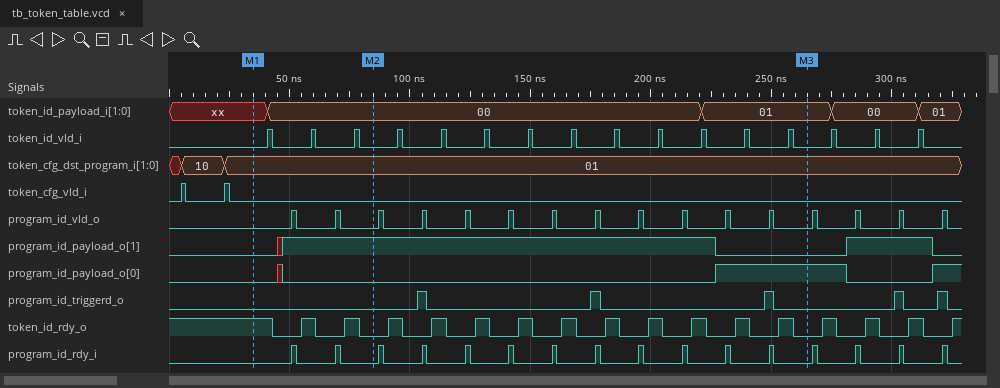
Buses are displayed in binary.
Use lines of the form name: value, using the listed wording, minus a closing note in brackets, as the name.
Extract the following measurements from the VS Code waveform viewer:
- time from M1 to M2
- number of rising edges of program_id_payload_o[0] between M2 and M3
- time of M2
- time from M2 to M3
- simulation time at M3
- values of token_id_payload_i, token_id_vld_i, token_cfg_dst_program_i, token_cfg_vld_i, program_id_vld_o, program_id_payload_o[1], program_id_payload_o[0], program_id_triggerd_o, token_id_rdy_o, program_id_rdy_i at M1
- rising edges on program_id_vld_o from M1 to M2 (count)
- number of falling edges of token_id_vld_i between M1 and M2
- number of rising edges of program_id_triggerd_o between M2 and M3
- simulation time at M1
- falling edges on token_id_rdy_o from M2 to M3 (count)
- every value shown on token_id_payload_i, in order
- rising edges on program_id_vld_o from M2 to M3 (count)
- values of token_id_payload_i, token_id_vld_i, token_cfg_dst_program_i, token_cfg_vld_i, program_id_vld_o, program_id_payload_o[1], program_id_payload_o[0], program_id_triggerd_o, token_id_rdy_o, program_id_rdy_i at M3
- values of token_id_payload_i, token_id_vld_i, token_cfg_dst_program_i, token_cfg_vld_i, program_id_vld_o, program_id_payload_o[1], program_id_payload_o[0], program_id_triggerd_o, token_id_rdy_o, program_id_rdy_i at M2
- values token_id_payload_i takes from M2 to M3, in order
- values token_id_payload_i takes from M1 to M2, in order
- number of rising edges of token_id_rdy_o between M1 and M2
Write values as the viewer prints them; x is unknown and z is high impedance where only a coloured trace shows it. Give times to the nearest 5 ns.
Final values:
time from M1 to M2: 50 ns
number of rising edges of program_id_payload_o[0] between M2 and M3: 1
time of M2: 85 ns
time from M2 to M3: 180 ns
simulation time at M3: 265 ns
values of token_id_payload_i, token_id_vld_i, token_cfg_dst_program_i, token_cfg_vld_i, program_id_vld_o, program_id_payload_o[1], program_id_payload_o[0], program_id_triggerd_o, token_id_rdy_o, program_id_rdy_i at M1: token_id_payload_i=xx, token_id_vld_i=0, token_cfg_dst_program_i=01, token_cfg_vld_i=0, program_id_vld_o=0, program_id_payload_o[1]=0, program_id_payload_o[0]=0, program_id_triggerd_o=0, token_id_rdy_o=1, program_id_rdy_i=0
rising edges on program_id_vld_o from M1 to M2: 2
number of falling edges of token_id_vld_i between M1 and M2: 3
number of rising edges of program_id_triggerd_o between M2 and M3: 3
simulation time at M1: 35 ns
falling edges on token_id_rdy_o from M2 to M3: 10
every value shown on token_id_payload_i, in order: xx, 00, 01, 00, 01
rising edges on program_id_vld_o from M2 to M3: 10
values of token_id_payload_i, token_id_vld_i, token_cfg_dst_program_i, token_cfg_vld_i, program_id_vld_o, program_id_payload_o[1], program_id_payload_o[0], program_id_triggerd_o, token_id_rdy_o, program_id_rdy_i at M3: token_id_payload_i=01, token_id_vld_i=0, token_cfg_dst_program_i=01, token_cfg_vld_i=0, program_id_vld_o=0, program_id_payload_o[1]=0, program_id_payload_o[0]=1, program_id_triggerd_o=0, token_id_rdy_o=0, program_id_rdy_i=0
values of token_id_payload_i, token_id_vld_i, token_cfg_dst_program_i, token_cfg_vld_i, program_id_vld_o, program_id_payload_o[1], program_id_payload_o[0], program_id_triggerd_o, token_id_rdy_o, program_id_rdy_i at M2: token_id_payload_i=00, token_id_vld_i=0, token_cfg_dst_program_i=01, token_cfg_vld_i=0, program_id_vld_o=0, program_id_payload_o[1]=1, program_id_payload_o[0]=0, program_id_triggerd_o=0, token_id_rdy_o=0, program_id_rdy_i=0
values token_id_payload_i takes from M2 to M3, in order: 00, 01
values token_id_payload_i takes from M1 to M2, in order: xx, 00
number of rising edges of token_id_rdy_o between M1 and M2: 2
